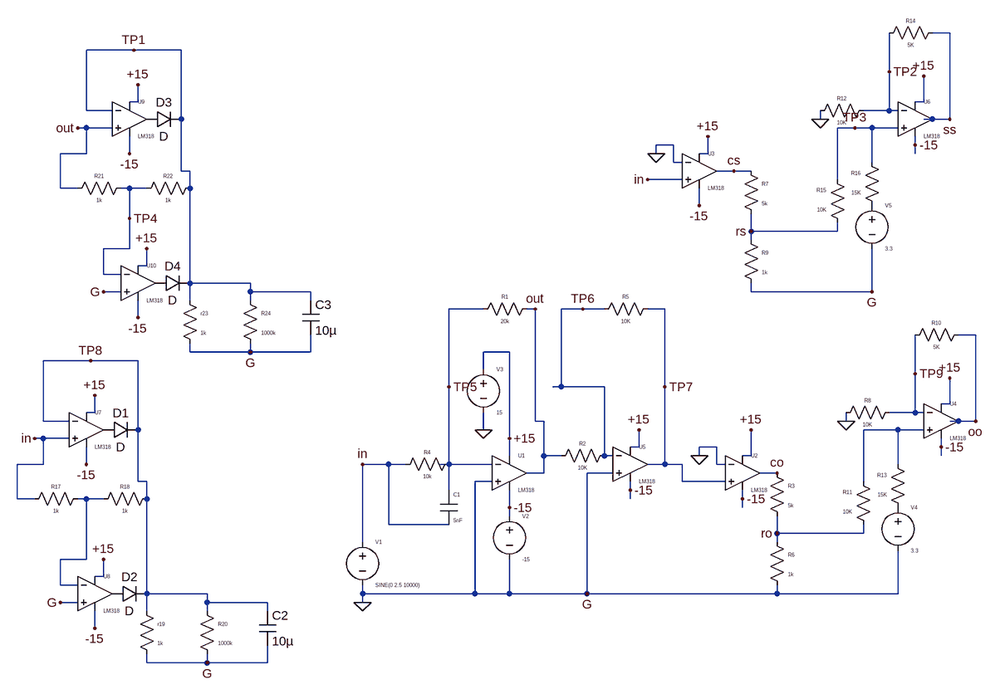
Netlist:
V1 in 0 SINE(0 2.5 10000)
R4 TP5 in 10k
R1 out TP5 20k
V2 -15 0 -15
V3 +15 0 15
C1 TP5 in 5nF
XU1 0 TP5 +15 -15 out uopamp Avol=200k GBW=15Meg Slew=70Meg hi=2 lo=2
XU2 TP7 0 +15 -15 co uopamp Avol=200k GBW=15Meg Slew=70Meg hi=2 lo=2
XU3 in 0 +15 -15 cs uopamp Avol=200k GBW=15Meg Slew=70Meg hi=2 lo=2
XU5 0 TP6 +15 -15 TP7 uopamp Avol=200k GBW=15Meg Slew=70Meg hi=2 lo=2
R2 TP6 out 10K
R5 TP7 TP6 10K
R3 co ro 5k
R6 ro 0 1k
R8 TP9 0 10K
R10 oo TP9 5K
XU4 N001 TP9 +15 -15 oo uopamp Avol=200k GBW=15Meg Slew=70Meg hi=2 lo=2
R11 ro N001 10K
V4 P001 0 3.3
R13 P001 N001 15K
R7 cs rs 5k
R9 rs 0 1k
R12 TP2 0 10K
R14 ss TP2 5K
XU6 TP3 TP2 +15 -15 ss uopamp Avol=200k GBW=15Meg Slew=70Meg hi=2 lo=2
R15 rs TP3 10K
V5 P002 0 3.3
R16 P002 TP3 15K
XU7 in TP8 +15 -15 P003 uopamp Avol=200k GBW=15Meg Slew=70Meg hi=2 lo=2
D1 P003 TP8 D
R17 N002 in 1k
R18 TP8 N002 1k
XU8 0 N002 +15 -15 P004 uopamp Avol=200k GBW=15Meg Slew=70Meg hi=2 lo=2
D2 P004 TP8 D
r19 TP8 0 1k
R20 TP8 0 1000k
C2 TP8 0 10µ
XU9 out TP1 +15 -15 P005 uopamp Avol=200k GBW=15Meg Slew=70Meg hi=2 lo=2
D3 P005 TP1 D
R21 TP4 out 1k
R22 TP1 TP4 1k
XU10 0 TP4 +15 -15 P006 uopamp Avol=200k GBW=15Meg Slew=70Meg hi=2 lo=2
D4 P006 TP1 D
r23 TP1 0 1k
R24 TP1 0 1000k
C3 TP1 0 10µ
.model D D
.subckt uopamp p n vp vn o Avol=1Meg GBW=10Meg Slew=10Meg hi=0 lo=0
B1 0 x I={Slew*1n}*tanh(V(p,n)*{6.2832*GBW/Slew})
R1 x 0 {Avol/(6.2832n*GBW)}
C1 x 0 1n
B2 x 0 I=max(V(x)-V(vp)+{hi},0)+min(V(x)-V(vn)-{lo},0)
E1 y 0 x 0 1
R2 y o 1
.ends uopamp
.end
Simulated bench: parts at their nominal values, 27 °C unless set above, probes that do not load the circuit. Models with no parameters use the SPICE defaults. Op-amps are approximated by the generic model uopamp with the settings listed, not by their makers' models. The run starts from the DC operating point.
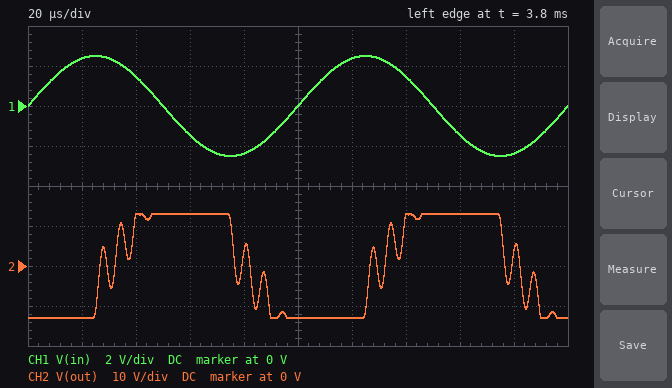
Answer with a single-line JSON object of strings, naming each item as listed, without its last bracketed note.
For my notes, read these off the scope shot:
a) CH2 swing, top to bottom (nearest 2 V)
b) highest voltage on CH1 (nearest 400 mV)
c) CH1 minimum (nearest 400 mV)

{"CH2 swing, top to bottom": "26 V", "highest voltage on CH1": "2.4 V", "CH1 minimum": "-2.4 V"}
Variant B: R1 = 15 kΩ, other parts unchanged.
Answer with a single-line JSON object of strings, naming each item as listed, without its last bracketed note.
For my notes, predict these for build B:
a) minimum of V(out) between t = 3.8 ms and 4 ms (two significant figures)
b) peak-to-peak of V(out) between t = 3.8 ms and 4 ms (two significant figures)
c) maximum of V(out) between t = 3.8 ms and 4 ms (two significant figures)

{"minimum of V(out) between t = 3.8 ms and 4 ms": "-12 V", "peak-to-peak of V(out) between t = 3.8 ms and 4 ms": "25 V", "maximum of V(out) between t = 3.8 ms and 4 ms": "12 V"}
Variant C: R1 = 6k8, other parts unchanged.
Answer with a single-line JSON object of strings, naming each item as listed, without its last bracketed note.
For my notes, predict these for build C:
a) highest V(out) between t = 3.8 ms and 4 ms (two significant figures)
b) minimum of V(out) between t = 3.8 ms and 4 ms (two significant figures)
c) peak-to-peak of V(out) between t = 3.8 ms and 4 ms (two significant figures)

{"highest V(out) between t = 3.8 ms and 4 ms": "5.6 V", "minimum of V(out) between t = 3.8 ms and 4 ms": "-5.6 V", "peak-to-peak of V(out) between t = 3.8 ms and 4 ms": "11 V"}
